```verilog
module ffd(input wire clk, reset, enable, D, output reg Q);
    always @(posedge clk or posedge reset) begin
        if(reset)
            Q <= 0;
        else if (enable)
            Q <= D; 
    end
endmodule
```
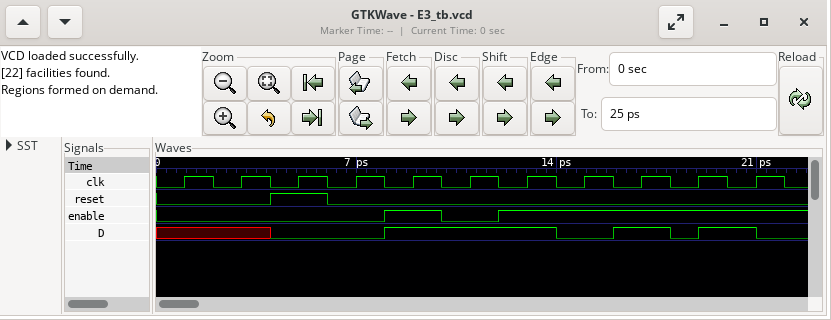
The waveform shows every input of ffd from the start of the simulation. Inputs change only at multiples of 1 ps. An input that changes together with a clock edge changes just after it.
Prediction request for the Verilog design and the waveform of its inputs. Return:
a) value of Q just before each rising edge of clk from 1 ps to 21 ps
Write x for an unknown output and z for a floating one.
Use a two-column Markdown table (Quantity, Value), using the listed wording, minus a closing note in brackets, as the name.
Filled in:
| Quantity | Value |
|---|---|
| value of Q just before each rising edge of clk from 1 ps to 21 ps | x x 0 0 0 1 1 1 0 1 0 |
